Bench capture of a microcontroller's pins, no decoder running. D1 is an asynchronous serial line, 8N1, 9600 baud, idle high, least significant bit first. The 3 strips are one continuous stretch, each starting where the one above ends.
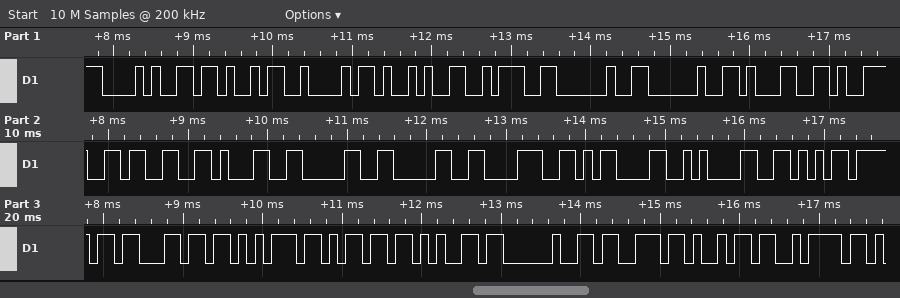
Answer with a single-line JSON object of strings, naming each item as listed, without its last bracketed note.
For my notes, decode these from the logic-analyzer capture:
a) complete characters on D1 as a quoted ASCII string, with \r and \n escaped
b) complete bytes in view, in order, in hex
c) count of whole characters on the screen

{"complete characters on D1 as a quoted ASCII string, with \\r and \\n escaped": "\"(KB):  1931008\\r\\nVolume siz\"", "complete bytes in view, in order, in hex": "28 4B 42 29 3A 20 20 31 39 33 31 30 30 38 0D 0A 56 6F 6C 75 6D 65 20 73 69 7A", "count of whole characters on the screen": "26"}
